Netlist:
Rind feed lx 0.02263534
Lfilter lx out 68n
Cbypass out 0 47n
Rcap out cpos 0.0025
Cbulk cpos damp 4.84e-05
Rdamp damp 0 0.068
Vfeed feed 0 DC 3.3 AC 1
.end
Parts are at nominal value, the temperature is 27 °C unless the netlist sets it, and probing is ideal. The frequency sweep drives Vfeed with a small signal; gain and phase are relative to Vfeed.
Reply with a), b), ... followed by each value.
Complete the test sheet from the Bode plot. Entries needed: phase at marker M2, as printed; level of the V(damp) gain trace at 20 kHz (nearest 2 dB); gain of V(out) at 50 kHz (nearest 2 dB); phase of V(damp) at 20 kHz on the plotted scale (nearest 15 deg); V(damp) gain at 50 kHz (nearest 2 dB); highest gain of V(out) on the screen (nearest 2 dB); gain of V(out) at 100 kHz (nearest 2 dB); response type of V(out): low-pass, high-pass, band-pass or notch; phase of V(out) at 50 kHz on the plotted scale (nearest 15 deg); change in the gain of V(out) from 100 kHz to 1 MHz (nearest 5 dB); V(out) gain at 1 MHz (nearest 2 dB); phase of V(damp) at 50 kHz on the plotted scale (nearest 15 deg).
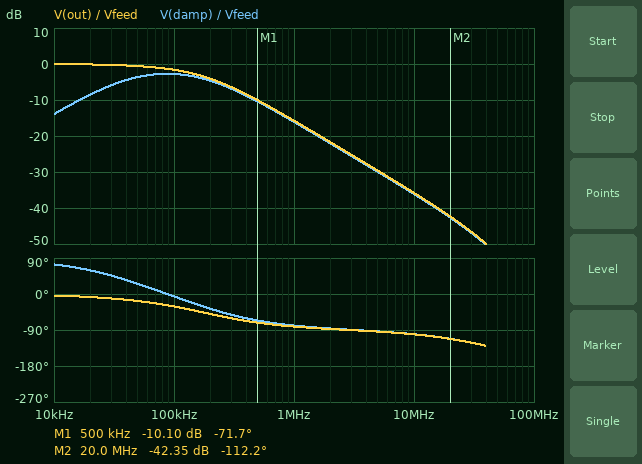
a) -112.2 deg
b) -8 dB
c) 0 dB
d) 60 deg
e) -4 dB
f) 0 dB
g) -2 dB
h) low-pass
i) -15 deg
j) -15 dB
k) -16 dB
l) 30 deg
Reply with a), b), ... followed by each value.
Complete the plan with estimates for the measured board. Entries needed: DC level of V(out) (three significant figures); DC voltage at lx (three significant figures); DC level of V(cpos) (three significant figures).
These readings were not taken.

a) 3.30 V
b) 3.30 V
c) 3.30 V
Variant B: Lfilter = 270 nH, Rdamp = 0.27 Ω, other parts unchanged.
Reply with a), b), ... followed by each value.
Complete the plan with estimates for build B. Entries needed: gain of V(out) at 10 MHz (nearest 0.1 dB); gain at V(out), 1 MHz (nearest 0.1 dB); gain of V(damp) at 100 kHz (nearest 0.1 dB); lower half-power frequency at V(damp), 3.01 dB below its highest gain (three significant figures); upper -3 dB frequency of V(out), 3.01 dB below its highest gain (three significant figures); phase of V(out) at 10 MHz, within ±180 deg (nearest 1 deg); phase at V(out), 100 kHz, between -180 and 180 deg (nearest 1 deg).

a) -38.0 dB
b) -15.9 dB
c) -1.6 dB
d) 10.5 kHz
e) 161 kHz
f) -128 deg
g) -32 deg
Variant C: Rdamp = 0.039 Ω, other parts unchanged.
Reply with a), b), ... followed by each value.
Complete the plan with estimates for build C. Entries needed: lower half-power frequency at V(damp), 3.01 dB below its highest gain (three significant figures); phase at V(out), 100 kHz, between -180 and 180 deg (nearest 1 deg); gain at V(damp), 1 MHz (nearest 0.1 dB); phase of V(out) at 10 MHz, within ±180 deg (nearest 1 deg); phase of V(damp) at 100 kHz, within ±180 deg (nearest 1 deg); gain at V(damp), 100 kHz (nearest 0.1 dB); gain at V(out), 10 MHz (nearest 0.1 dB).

a) 40.4 kHz
b) -47 deg
c) -20.8 dB
d) -97 deg
e) -9 deg
f) -4.4 dB
g) -40.3 dB
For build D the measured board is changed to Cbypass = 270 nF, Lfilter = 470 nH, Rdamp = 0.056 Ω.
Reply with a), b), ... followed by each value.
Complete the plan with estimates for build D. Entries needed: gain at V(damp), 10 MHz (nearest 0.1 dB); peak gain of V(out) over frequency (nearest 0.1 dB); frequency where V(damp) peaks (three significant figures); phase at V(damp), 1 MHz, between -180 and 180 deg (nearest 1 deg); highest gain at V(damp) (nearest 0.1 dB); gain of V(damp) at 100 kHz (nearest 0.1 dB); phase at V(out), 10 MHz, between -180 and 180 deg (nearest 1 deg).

a) -57.4 dB
b) 3.5 dB
c) 33.3 kHz
d) -94 deg
e) -3.2 dB
f) -13.8 dB
g) -135 deg
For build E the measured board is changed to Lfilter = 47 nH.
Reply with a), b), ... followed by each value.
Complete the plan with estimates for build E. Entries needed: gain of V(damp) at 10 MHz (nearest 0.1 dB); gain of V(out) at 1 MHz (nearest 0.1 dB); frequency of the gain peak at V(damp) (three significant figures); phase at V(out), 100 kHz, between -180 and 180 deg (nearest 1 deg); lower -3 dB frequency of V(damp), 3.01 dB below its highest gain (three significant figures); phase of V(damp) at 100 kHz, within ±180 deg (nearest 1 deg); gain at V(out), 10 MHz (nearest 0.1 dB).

a) -32.9 dB
b) -12.7 dB
c) 106 kHz
d) -23 deg
e) 32.1 kHz
f) 2 deg
g) -32.6 dB
